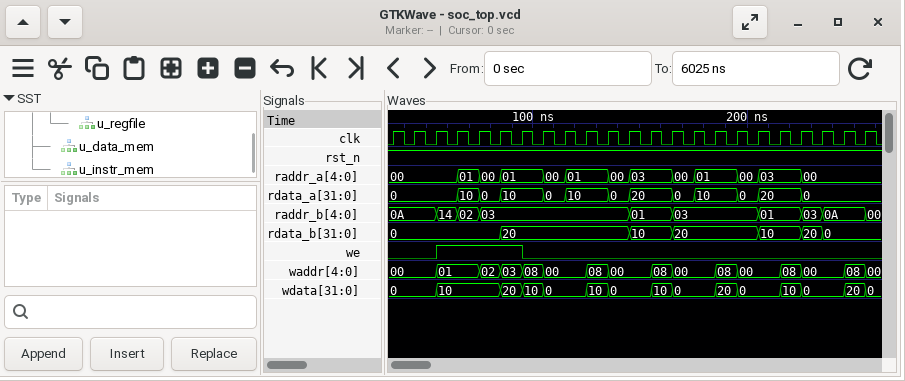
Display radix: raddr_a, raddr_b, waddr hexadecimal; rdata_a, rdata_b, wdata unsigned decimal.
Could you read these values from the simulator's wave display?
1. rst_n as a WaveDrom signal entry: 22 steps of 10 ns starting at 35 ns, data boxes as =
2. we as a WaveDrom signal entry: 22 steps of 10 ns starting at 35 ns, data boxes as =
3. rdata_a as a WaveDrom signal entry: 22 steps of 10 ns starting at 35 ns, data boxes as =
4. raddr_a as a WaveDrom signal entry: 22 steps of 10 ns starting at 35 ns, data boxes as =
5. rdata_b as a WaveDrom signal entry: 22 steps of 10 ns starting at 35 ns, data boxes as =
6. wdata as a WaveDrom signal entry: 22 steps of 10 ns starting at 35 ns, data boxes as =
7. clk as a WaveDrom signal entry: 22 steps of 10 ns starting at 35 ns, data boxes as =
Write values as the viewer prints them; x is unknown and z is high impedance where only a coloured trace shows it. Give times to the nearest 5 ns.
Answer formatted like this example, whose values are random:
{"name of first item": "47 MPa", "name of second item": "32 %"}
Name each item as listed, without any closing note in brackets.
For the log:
{"rst_n as a WaveDrom signal entry: 22 steps of 10 ns starting at 35 ns, data boxes as =": "{name: 'rst_n', wave: '1.....................'}", "we as a WaveDrom signal entry: 22 steps of 10 ns starting at 35 ns, data boxes as =": "{name: 'we', wave: '0.1...0...............'}", "rdata_a as a WaveDrom signal entry: 22 steps of 10 ns starting at 35 ns, data boxes as =": "{name: 'rdata_a', wave: '=..===.==.==.==.==.=..', data: '0 10 0 10 0 10 0 20 0 10 0 20 0'}", "raddr_a as a WaveDrom signal entry: 22 steps of 10 ns starting at 35 ns, data boxes as =": "{name: 'raddr_a', wave: '=..===.==.==.==.==.=..', data: '00 01 00 01 00 01 00 03 00 01 00 03 00'}", "rdata_b as a WaveDrom signal entry: 22 steps of 10 ns starting at 35 ns, data boxes as =": "{name: 'rdata_b', wave: '=....=.....=.=...=.==.', data: '0 20 10 20 10 20 0'}", "wdata as a WaveDrom signal entry: 22 steps of 10 ns starting at 35 ns, data boxes as =": "{name: 'wdata', wave: '=.=..===.==.==.==.==.=', data: '0 10 20 10 0 10 0 10 0 20 0 10 0 20'}", "clk as a WaveDrom signal entry: 22 steps of 10 ns starting at 35 ns, data boxes as =": "{name: 'clk', wave: 'p.....................'}"}
